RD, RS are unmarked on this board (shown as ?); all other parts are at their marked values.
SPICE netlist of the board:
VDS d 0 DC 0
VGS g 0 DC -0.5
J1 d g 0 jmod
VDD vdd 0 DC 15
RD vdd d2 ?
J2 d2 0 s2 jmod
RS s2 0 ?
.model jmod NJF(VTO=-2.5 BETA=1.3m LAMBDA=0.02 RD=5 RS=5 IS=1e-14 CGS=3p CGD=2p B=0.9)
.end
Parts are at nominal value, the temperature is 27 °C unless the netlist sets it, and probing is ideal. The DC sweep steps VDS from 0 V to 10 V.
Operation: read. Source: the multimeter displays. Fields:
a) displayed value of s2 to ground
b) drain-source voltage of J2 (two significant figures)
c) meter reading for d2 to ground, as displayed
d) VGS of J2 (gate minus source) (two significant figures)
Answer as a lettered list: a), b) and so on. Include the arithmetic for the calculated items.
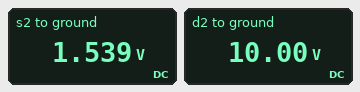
a) 1.539 V
b) 10 V - 1.539 V = 8.5 V
c) 10.00 V
d) 0 V - 1.539 V = -1.5 V
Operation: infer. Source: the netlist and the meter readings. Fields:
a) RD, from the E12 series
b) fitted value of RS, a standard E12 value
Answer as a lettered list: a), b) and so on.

a) 3.9 kΩ
b) 1.2 kΩ
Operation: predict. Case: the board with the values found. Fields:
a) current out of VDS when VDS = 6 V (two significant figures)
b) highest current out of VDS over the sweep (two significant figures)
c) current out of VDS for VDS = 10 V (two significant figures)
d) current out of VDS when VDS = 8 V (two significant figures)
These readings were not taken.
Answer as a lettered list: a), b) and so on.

a) 5.4 mA
b) 5.8 mA
c) 5.8 mA
d) 5.6 mA
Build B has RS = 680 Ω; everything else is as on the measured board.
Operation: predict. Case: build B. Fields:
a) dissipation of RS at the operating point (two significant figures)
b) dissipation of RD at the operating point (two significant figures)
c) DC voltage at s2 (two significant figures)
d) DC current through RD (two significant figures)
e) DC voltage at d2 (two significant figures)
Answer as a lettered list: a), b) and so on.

a) 2.5 mW
b) 14 mW
c) 1.3 V
d) 1.9 mA
e) 7.5 V
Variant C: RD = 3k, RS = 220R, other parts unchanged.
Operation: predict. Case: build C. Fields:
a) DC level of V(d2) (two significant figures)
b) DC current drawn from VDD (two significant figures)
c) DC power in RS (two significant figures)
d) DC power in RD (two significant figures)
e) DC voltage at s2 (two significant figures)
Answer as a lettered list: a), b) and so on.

a) 4.0 V
b) 3.7 mA
c) 3.0 mW
d) 40 mW
e) 810 mV
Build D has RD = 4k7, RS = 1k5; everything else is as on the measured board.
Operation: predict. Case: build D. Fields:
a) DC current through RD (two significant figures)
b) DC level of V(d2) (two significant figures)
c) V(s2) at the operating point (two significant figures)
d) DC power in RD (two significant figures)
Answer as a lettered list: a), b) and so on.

a) 1.1 mA
b) 9.9 V
c) 1.6 V
d) 5.5 mW
